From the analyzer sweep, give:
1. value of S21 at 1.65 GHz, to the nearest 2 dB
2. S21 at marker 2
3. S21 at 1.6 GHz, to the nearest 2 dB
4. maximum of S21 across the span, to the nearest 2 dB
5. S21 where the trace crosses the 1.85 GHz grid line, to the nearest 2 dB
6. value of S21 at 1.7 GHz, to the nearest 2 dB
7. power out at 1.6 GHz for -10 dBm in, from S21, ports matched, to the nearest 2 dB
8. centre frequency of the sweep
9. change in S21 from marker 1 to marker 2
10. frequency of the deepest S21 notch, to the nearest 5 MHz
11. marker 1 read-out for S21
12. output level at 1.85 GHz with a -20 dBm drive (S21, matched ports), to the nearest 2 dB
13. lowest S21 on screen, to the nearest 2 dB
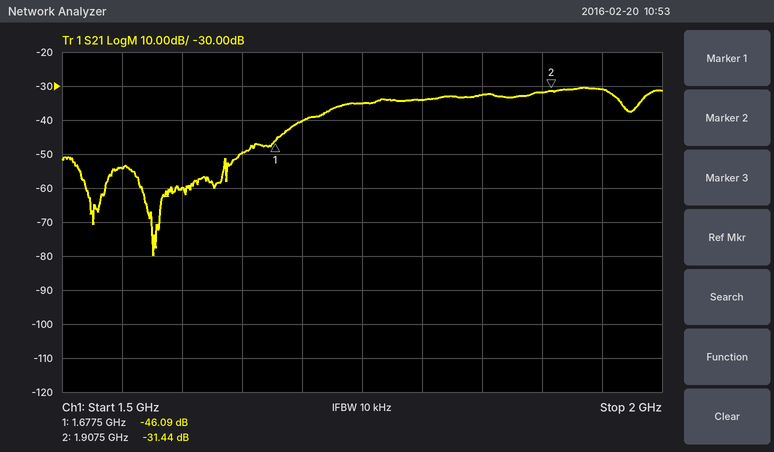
-50 dB
-31.44 dB
-60 dB
-30 dB
-32 dB
-40 dB
-70 dBm
1.75 GHz
14.65 dB
1.575 GHz
-46.09 dB
-52 dBm
-80 dB
